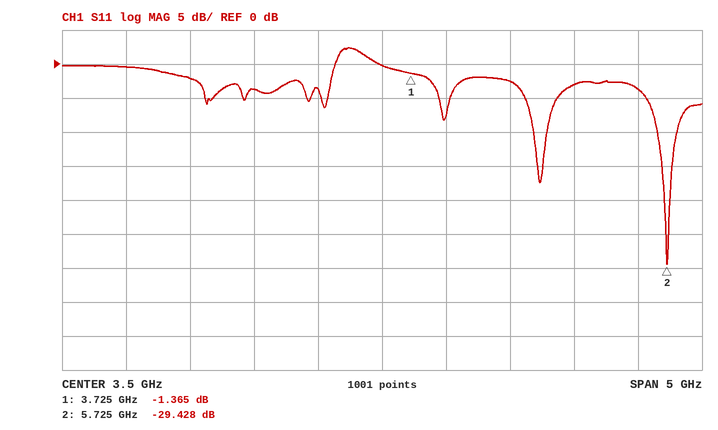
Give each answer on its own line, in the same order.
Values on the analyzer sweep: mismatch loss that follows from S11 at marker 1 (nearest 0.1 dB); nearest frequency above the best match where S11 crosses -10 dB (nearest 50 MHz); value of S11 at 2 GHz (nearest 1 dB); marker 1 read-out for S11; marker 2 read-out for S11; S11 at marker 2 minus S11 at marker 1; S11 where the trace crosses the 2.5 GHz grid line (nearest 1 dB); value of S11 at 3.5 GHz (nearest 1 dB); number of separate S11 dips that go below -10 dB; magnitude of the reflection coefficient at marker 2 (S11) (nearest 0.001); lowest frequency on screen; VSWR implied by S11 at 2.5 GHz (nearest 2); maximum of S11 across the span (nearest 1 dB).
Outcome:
5.7 dB
5.80 GHz
-2 dB
-1.365 dB
-29.428 dB
-28.063 dB
-4 dB
0 dB
2
0.034
1 GHz
4
2 dB
